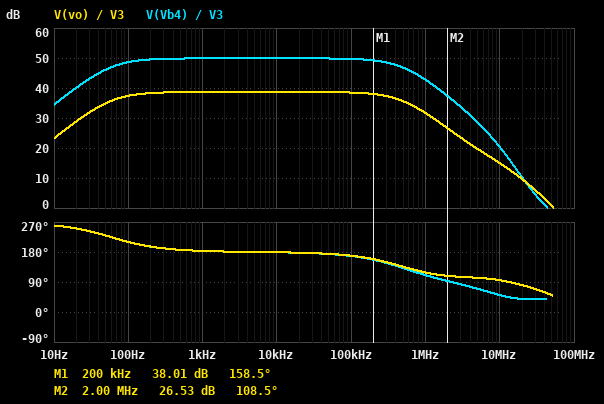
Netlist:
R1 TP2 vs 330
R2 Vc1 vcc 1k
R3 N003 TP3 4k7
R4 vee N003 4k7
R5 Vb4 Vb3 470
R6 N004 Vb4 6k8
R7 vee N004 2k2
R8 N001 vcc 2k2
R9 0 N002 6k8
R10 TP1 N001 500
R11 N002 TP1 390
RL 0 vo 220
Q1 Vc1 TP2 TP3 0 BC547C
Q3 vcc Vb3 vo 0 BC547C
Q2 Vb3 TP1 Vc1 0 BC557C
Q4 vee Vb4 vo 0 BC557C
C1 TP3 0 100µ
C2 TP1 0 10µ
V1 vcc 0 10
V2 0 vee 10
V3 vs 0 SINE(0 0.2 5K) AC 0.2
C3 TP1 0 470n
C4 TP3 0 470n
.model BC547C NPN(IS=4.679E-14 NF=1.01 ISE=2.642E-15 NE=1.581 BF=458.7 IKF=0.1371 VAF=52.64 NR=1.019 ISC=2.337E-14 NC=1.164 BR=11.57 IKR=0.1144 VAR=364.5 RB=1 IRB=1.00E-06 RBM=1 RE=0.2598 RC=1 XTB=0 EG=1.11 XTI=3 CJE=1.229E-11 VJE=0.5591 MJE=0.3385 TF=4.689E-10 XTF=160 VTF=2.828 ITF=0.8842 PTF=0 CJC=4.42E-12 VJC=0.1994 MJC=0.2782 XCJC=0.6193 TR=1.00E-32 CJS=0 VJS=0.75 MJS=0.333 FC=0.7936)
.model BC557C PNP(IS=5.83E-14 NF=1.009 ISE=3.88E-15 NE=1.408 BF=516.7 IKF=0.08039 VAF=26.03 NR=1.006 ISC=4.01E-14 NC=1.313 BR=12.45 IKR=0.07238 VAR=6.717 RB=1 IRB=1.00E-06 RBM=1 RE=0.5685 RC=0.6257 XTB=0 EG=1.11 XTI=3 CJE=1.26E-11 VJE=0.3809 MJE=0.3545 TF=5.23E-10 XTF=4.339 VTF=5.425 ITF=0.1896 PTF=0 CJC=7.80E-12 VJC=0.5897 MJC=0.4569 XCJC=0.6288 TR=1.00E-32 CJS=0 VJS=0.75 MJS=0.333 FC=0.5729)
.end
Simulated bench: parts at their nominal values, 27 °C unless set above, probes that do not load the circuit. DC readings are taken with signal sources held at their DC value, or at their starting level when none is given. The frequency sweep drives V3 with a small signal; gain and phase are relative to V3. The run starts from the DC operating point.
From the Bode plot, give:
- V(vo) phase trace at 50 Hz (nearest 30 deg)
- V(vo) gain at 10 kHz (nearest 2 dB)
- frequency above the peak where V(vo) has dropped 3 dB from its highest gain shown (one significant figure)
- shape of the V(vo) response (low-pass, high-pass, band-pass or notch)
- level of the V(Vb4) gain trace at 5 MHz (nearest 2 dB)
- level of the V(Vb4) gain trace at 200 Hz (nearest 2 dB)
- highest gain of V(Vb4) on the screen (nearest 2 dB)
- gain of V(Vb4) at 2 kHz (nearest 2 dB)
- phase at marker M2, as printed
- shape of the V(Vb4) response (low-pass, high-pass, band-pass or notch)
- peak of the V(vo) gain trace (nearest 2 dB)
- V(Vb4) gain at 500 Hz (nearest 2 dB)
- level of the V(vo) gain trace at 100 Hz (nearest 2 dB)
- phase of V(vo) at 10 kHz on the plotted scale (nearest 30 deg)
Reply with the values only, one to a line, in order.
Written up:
240 deg
38 dB
500 kHz
band-pass
28 dB
50 dB
50 dB
50 dB
108.5 deg
band-pass
38 dB
50 dB
38 dB
180 deg
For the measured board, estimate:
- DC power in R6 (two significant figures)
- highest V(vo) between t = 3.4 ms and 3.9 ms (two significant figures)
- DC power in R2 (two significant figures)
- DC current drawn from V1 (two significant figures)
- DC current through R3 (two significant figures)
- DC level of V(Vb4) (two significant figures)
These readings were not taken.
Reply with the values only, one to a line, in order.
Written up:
8.4 mW
7.2 V
4.5 mW
3.2 mA
1.0 mA
20 mV
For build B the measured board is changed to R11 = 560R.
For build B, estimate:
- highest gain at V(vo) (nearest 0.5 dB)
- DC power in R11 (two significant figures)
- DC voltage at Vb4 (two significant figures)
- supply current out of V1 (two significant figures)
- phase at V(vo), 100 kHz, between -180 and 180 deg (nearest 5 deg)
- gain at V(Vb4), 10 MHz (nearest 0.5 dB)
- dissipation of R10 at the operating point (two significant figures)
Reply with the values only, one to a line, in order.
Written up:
16.0 dB
550 µW
-380 mV
3.1 mA
-120 deg
18.5 dB
490 µW
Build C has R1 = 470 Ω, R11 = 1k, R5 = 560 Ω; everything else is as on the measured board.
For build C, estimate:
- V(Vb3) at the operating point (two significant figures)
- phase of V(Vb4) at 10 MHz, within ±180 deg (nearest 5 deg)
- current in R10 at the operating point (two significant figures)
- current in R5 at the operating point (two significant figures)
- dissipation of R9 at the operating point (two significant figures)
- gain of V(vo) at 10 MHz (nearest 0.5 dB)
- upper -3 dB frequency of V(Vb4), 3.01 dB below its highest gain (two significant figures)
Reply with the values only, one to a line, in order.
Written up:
-770 mV
25 deg
950 µA
960 µA
6.2 mW
28.5 dB
1.7 MHz
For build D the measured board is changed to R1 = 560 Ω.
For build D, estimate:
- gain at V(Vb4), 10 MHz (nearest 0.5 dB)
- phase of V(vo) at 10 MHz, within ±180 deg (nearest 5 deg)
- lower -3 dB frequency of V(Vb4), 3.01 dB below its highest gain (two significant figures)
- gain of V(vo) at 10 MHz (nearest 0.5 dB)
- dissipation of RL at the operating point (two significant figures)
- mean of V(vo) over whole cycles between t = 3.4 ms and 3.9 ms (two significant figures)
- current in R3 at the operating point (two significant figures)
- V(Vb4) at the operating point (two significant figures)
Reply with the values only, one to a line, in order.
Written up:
17.5 dB
80 deg
57 Hz
12.0 dB
400 nW
1.7 V
1.0 mA
21 mV
